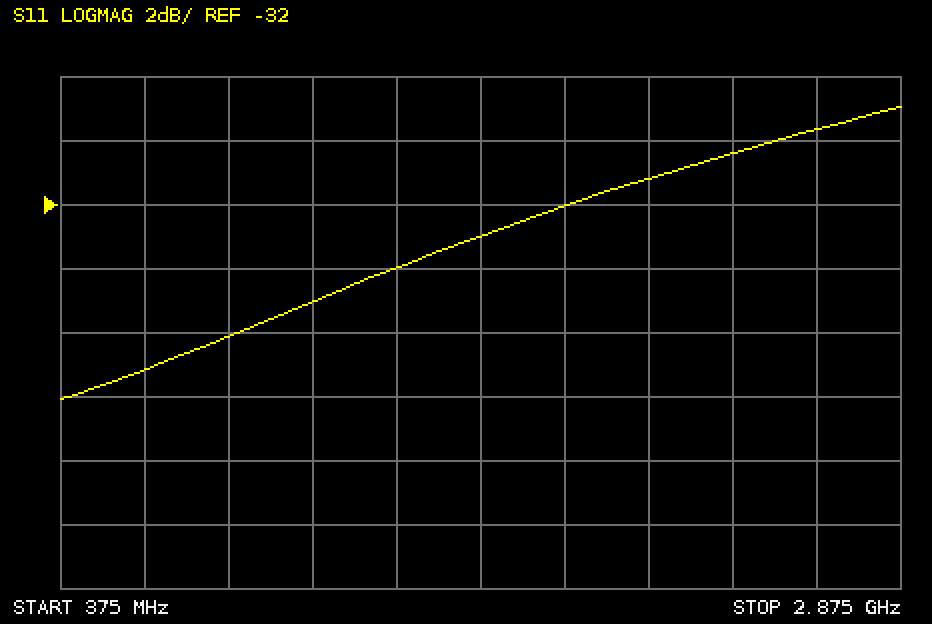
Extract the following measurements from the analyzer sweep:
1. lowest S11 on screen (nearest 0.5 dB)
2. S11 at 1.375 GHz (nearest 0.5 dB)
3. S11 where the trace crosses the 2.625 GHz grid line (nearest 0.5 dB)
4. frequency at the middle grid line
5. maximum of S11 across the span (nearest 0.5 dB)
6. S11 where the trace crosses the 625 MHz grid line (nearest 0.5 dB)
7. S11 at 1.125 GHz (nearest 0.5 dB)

-38.0 dB
-34.0 dB
-29.5 dB
1.625 GHz
-29.0 dB
-37.0 dB
-35.0 dB
